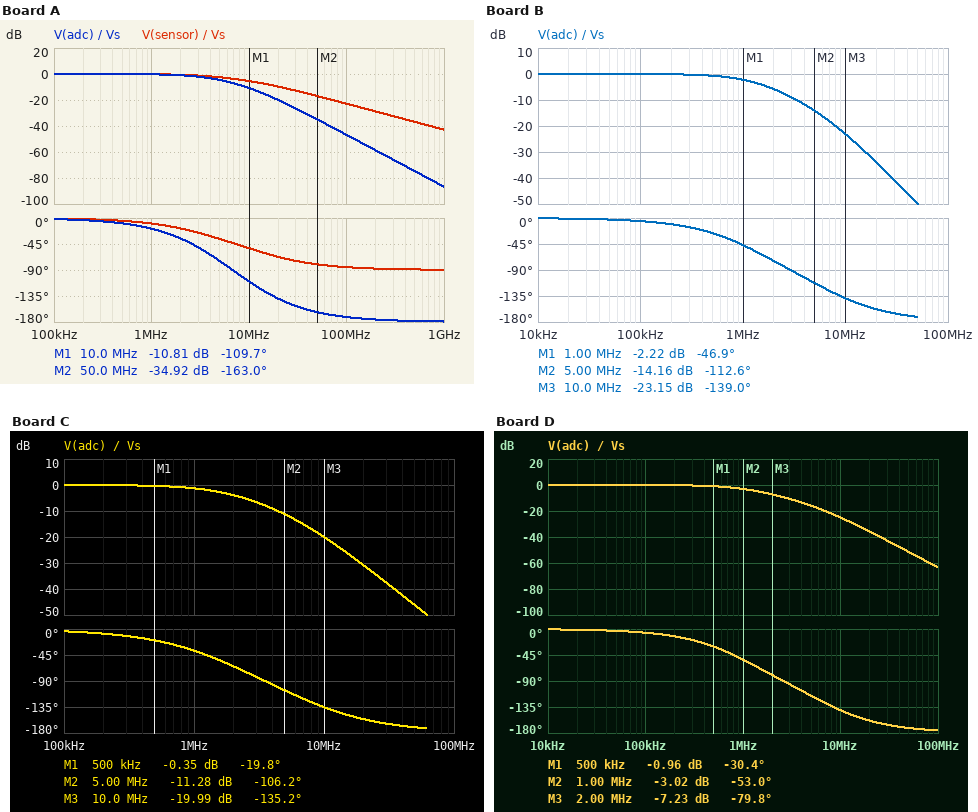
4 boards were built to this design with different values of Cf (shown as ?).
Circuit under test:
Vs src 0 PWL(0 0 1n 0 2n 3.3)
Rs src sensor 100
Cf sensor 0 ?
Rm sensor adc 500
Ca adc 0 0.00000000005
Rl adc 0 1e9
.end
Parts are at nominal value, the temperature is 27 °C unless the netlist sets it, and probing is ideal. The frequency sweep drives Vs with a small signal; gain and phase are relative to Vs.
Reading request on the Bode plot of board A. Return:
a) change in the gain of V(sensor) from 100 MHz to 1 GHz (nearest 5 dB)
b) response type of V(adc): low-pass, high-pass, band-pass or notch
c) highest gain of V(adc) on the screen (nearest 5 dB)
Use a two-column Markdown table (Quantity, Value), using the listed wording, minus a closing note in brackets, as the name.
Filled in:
| Quantity | Value |
|---|---|
| change in the gain of V(sensor) from 100 MHz to 1 GHz | -20 dB |
| response type of V(adc): low-pass, high-pass, band-pass or notch | low-pass |
| highest gain of V(adc) on the screen | 0 dB |
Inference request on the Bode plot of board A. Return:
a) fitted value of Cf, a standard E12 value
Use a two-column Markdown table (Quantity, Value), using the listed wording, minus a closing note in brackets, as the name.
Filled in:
| Quantity | Value |
|---|---|
| fitted value of Cf, a standard E12 value | 220 pF |
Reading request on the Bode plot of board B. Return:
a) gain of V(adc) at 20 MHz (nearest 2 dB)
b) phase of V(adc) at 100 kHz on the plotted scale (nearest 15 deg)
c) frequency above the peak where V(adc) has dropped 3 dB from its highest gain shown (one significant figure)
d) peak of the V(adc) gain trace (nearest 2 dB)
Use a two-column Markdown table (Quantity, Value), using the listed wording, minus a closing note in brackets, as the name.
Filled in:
| Quantity | Value |
|---|---|
| gain of V(adc) at 20 MHz | -34 dB |
| phase of V(adc) at 100 kHz on the plotted scale | 0 deg |
| frequency above the peak where V(adc) has dropped 3 dB from its highest gain shown | 1 MHz |
| peak of the V(adc) gain trace | 0 dB |
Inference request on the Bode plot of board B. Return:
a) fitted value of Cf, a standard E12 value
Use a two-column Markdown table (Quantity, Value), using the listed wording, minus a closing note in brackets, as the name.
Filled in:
| Quantity | Value |
|---|---|
| fitted value of Cf, a standard E12 value | 1.2 nF |
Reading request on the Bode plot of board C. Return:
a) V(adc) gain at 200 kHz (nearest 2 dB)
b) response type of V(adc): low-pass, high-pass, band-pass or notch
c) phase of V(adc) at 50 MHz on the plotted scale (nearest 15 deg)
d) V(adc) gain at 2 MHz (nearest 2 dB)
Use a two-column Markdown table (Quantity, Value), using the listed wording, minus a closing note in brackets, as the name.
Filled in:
| Quantity | Value |
|---|---|
| V(adc) gain at 200 kHz | 0 dB |
| response type of V(adc): low-pass, high-pass, band-pass or notch | low-pass |
| phase of V(adc) at 50 MHz on the plotted scale | -165 deg |
| V(adc) gain at 2 MHz | -4 dB |
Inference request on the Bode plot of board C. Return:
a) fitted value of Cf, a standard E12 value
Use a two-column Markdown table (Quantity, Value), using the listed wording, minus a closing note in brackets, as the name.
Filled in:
| Quantity | Value |
|---|---|
| fitted value of Cf, a standard E12 value | 820 pF |
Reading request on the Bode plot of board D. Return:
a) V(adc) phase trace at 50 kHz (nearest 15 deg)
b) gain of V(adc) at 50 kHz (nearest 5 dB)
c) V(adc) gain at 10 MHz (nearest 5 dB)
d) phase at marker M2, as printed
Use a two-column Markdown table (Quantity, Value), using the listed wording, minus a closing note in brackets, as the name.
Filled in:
| Quantity | Value |
|---|---|
| V(adc) phase trace at 50 kHz | 0 deg |
| gain of V(adc) at 50 kHz | 0 dB |
| V(adc) gain at 10 MHz | -25 dB |
| phase at marker M2, as printed | -53.0 deg |
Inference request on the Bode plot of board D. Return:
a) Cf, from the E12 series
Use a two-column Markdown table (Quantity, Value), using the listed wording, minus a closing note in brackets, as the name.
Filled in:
| Quantity | Value |
|---|---|
| Cf, from the E12 series | 1.5 nF |
